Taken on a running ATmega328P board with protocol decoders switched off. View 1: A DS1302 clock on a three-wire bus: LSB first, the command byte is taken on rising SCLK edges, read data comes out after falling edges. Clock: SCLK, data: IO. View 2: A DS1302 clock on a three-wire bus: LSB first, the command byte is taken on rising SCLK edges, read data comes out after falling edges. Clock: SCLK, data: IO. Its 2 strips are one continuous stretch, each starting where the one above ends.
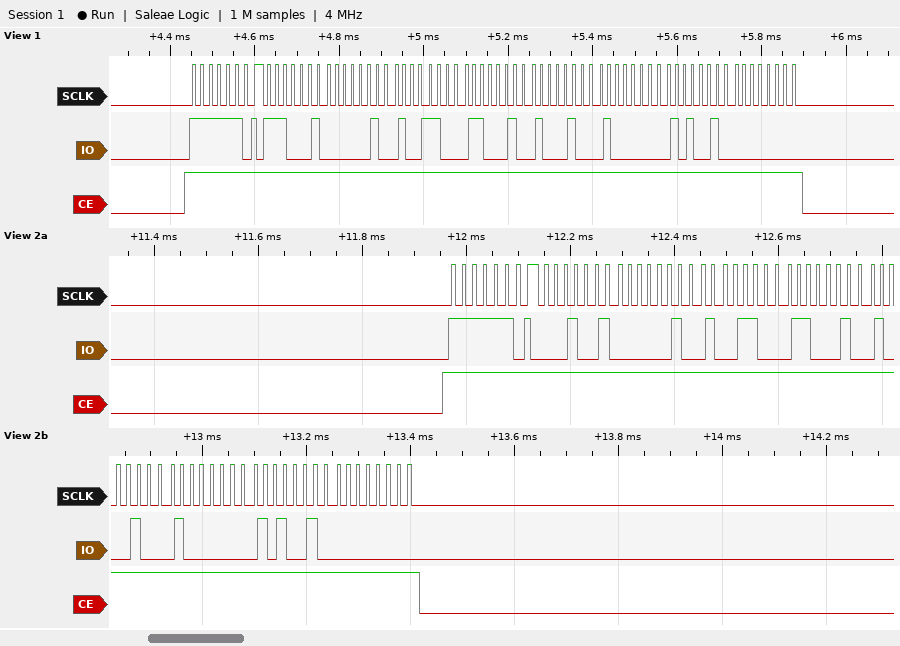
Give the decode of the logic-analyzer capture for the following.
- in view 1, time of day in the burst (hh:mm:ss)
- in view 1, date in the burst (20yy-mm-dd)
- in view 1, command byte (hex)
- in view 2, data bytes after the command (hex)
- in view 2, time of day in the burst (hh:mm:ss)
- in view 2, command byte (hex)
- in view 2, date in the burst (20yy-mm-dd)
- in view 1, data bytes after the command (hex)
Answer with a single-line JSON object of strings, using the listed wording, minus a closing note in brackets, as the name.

{"in view 1, time of day in the burst": "19:20:47", "in view 1, date in the burst": "2025-11-23", "in view 1, command byte": "0xBF", "in view 2, data bytes after the command": "48 20 19 23 11 01 25 00", "in view 2, time of day in the burst": "19:20:48", "in view 2, command byte": "0xBF", "in view 2, date in the burst": "2025-11-23", "in view 1, data bytes after the command": "47 20 19 23 11 01 25 00"}
